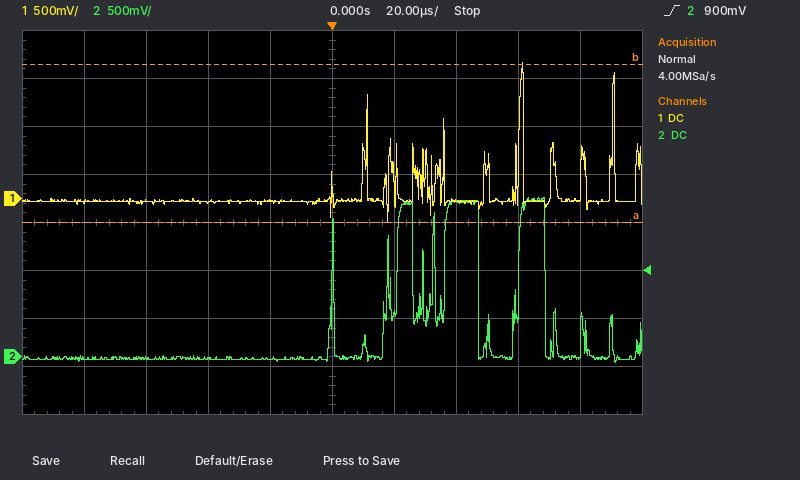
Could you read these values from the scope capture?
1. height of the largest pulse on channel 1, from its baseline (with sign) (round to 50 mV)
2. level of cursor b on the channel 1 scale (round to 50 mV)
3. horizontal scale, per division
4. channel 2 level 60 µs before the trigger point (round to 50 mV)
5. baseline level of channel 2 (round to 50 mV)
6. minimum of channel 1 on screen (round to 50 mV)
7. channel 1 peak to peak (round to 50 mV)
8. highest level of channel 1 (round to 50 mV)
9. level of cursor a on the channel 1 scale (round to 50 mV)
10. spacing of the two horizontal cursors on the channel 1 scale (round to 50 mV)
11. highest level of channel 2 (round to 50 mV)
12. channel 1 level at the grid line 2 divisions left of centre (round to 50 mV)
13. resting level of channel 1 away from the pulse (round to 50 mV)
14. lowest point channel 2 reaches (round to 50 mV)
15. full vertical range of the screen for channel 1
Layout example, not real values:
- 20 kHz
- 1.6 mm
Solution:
- +1.45 V
- 1.40 V
- 20 µs
- 0 mV
- 0 mV
- -250 mV
- 1.65 V
- 1.40 V
- -250 mV
- 1.65 V
- 1.65 V
- -50 mV
- -50 mV
- -50 mV
- 4 V
